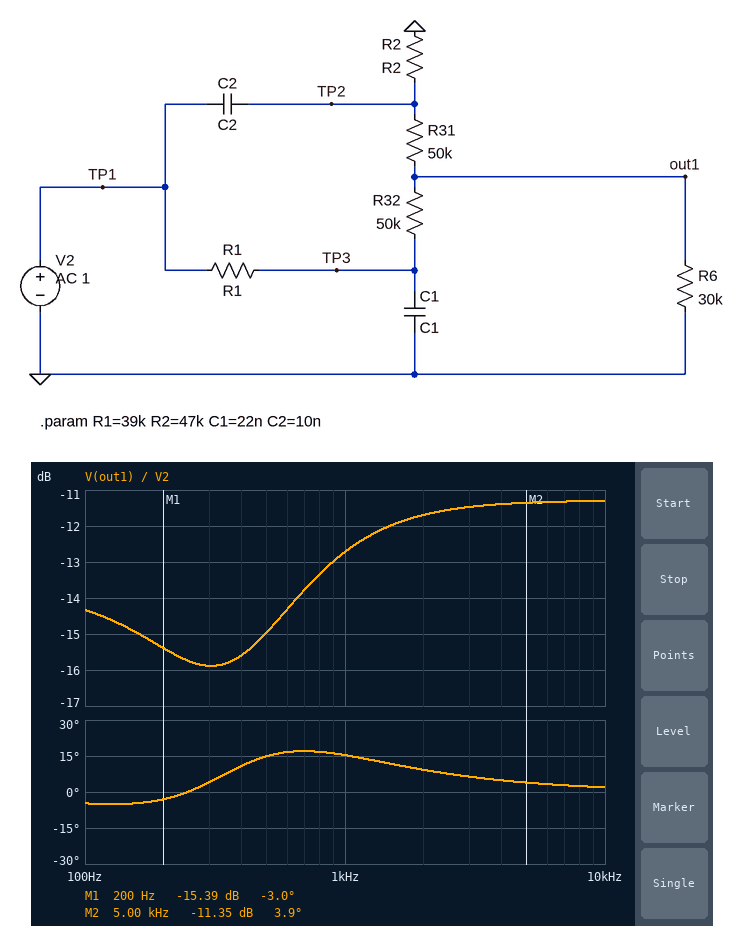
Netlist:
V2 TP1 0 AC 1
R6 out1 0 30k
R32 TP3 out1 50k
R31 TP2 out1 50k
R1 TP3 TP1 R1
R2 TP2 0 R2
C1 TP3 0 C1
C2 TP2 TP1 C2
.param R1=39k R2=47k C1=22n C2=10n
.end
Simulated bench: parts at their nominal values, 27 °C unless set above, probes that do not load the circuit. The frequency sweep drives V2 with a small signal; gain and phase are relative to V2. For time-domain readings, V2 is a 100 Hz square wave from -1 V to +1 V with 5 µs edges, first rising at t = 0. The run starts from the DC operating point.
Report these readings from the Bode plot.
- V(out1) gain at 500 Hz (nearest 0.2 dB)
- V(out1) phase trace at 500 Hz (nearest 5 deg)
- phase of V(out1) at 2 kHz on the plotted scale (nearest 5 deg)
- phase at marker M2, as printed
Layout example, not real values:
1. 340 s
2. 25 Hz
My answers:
1. -15.0 dB
2. 15 deg
3. 10 deg
4. 3.9 deg
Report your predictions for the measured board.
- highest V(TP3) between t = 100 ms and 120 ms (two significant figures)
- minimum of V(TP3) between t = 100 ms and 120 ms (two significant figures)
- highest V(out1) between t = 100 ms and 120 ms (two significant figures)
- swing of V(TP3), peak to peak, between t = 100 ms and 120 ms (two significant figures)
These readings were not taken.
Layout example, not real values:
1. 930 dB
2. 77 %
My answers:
1. 650 mV
2. -650 mV
3. 340 mV
4. 1.3 V
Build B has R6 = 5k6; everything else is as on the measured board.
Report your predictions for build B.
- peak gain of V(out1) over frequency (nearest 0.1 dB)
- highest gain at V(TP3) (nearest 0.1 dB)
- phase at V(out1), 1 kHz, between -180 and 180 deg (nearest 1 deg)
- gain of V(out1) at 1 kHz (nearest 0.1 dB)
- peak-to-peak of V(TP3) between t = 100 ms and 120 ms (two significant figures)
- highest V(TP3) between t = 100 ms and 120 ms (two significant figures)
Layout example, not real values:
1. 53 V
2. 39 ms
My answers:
1. -20.8 dB
2. -4.6 dB
3. 19 deg
4. -22.5 dB
5. 1.2 V
6. 590 mV
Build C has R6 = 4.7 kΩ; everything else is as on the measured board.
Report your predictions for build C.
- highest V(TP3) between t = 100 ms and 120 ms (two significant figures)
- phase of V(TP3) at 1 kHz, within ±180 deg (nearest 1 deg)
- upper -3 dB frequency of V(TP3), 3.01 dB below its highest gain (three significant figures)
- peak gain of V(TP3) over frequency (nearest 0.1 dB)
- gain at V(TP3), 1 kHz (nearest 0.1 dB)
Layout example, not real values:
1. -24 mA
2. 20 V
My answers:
1. 580 mV
2. -71 deg
3. 326 Hz
4. -4.7 dB
5. -14.7 dB
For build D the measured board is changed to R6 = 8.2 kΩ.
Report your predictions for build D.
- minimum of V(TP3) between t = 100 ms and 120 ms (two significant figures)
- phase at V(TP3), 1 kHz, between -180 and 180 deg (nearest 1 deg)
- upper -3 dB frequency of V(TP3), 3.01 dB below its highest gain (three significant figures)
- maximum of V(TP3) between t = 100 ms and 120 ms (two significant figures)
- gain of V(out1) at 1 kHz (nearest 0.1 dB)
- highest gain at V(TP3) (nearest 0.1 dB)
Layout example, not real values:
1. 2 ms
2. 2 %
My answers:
1. -600 mV
2. -70 deg
3. 324 Hz
4. 600 mV
5. -19.8 dB
6. -4.5 dB
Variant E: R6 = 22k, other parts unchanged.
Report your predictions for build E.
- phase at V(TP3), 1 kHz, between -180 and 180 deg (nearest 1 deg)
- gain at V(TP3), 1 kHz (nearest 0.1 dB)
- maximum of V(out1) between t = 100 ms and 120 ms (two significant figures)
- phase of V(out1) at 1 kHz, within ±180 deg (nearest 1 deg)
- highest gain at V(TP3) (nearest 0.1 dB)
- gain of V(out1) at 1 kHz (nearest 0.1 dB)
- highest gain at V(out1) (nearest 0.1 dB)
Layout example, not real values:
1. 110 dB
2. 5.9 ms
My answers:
1. -70 deg
2. -13.9 dB
3. 300 mV
4. 16 deg
5. -3.9 dB
6. -14.1 dB
7. -12.6 dB
